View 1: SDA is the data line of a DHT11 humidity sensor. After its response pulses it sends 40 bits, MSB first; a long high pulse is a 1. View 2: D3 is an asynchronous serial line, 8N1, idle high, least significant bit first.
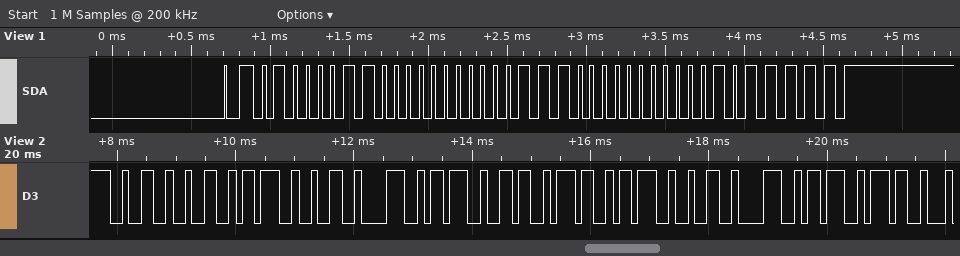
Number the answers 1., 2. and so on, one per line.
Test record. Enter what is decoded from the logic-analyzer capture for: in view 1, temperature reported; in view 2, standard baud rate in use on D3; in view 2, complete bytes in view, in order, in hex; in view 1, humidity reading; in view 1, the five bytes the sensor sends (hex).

1. 28.0 °C
2. 9600 baud
3. 32 32 3B 32 38 3B 36 37 3B 32 38 3B 37
4. 67 %
5. 43 00 1C 00 5F
